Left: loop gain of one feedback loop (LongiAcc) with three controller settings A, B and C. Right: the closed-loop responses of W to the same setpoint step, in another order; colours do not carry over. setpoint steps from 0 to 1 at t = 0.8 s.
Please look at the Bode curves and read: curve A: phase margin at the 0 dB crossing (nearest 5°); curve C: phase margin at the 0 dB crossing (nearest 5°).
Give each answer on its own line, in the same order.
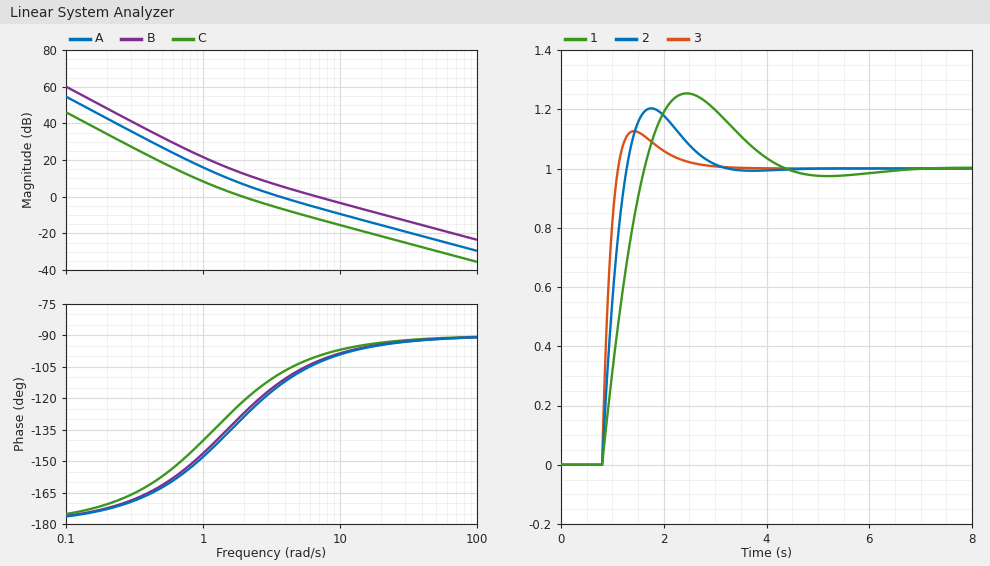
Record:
65°
60°
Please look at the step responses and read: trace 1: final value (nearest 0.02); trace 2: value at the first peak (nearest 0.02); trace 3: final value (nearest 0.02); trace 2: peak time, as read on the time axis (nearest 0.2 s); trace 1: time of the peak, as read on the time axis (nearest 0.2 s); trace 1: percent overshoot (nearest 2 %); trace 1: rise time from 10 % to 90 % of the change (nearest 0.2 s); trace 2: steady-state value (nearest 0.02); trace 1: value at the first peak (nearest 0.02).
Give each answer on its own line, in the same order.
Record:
1.00
1.20
1.00
1.8 s
2.4 s
26 %
0.6 s
1.00
1.26
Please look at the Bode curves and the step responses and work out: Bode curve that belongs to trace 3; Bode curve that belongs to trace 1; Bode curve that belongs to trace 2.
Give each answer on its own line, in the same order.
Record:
B
C
A
